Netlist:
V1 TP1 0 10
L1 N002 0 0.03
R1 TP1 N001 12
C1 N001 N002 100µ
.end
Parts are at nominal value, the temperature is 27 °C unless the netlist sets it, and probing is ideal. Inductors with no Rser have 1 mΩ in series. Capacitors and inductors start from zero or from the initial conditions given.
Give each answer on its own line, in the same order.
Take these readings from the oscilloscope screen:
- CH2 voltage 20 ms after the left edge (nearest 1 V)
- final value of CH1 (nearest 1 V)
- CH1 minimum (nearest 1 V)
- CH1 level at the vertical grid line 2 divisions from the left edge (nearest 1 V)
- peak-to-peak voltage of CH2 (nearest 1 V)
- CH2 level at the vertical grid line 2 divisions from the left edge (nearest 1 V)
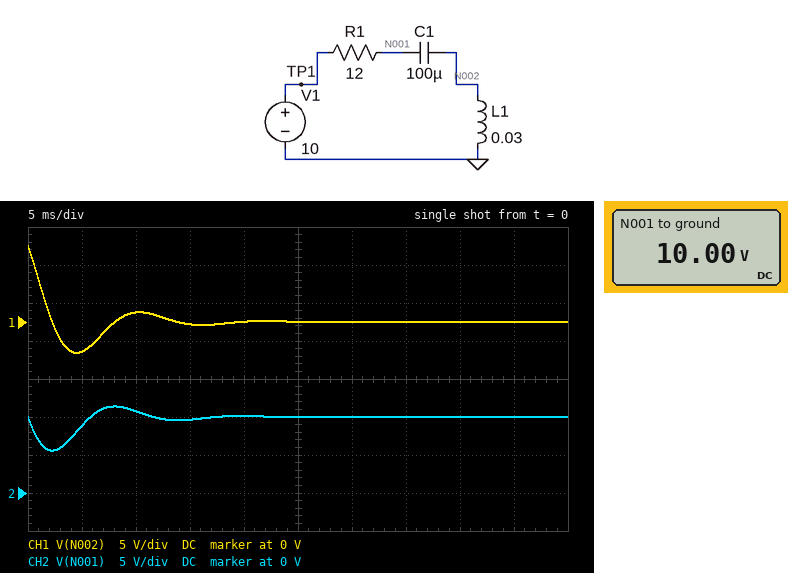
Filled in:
10 V
0 V
-4 V
1 V
6 V
11 V
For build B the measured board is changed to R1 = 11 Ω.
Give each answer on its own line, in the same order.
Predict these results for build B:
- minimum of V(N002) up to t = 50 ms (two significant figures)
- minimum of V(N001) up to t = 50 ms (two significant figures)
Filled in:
-4.3 V
5.8 V
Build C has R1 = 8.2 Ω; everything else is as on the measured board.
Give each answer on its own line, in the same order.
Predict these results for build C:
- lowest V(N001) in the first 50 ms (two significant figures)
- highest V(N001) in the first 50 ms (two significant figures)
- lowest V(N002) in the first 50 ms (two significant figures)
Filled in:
6.6 V
12 V
-5.2 V
